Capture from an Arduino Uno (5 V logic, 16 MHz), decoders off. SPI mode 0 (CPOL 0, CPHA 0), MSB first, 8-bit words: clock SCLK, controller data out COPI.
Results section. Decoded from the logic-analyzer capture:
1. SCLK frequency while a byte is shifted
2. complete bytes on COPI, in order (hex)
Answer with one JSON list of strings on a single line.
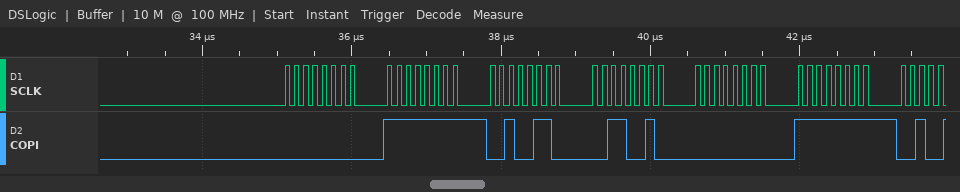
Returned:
["8 MHz", "00 FF 26 32 00 FF"]
